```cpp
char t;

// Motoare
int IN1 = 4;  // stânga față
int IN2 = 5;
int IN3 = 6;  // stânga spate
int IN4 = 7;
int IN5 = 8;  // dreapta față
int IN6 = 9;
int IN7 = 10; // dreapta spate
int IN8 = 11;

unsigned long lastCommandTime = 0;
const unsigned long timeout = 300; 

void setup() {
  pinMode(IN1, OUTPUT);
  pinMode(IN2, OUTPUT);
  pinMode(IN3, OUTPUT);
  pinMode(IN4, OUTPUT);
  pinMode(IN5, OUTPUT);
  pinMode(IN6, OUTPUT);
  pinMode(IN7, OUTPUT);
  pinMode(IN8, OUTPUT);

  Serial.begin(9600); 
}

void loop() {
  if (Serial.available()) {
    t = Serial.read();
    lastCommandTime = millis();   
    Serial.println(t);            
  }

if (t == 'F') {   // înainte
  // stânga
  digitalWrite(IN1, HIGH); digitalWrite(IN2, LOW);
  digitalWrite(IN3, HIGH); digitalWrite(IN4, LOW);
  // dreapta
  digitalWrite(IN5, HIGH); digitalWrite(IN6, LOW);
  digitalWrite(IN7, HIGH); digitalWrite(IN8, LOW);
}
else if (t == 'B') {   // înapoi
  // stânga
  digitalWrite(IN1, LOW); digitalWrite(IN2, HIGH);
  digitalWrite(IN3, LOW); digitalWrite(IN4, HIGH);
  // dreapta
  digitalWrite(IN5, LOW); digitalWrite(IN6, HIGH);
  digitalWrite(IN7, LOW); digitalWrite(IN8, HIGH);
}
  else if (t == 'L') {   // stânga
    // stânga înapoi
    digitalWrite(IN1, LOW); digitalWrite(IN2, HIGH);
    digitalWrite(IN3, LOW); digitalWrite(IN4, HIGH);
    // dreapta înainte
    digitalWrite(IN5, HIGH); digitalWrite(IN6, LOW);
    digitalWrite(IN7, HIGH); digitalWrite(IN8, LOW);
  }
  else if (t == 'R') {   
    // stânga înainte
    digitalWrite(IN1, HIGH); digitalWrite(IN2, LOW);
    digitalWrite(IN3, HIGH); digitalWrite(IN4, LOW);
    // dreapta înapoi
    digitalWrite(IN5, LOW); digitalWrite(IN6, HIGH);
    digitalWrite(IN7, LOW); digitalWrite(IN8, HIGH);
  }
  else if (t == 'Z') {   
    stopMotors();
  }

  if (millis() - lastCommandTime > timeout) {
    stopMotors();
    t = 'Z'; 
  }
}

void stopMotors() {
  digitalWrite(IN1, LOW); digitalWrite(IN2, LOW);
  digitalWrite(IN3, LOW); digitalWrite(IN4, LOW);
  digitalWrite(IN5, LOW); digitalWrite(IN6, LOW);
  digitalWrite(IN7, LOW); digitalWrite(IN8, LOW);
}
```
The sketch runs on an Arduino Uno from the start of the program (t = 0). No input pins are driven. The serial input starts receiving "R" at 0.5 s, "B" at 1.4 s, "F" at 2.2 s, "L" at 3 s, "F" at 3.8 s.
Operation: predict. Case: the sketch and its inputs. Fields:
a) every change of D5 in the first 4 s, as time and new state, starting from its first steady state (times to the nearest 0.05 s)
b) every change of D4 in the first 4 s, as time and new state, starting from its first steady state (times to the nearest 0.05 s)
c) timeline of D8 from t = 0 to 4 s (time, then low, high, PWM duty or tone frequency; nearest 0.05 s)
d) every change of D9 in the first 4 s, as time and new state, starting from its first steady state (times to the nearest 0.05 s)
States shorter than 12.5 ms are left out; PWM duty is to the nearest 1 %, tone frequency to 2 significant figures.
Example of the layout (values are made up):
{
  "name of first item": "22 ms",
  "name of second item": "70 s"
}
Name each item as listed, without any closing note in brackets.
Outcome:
{
  "every change of D5 in the first 4 s, as time and new state, starting from its first steady state": "0 s low; 1.4 s high; 1.7 s low; 3 s high; 3.3 s low",
  "every change of D4 in the first 4 s, as time and new state, starting from its first steady state": "0 s low; 0.5 s high; 0.8 s low; 2.2 s high; 2.5 s low; 3.8 s high",
  "timeline of D8 from t = 0 to 4 s": "0 s low; 2.2 s high; 2.5 s low; 3 s high; 3.3 s low; 3.8 s high",
  "every change of D9 in the first 4 s, as time and new state, starting from its first steady state": "0 s low; 0.5 s high; 0.8 s low; 1.4 s high; 1.7 s low"
}
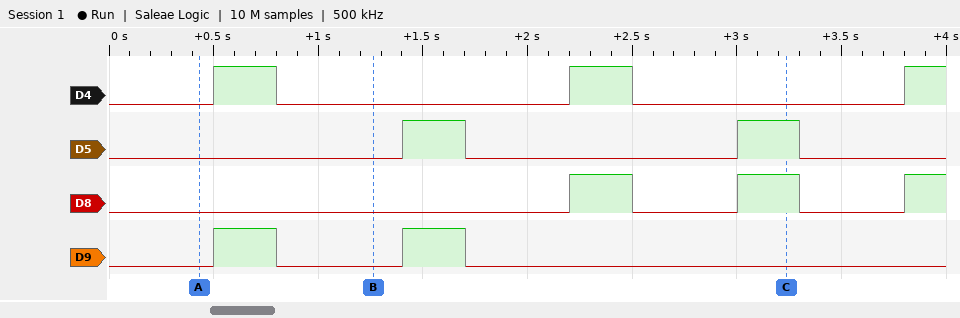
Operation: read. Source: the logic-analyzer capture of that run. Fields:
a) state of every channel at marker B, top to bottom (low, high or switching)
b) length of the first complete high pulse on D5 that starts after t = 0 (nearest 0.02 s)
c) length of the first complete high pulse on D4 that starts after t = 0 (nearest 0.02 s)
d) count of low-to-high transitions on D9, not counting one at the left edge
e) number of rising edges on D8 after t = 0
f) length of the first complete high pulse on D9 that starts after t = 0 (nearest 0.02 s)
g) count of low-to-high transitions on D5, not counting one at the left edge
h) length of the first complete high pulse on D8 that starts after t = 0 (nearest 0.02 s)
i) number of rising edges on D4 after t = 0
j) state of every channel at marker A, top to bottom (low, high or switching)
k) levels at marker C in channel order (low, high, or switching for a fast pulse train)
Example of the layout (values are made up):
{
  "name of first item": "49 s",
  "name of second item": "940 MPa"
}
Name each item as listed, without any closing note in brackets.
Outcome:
{
  "state of every channel at marker B, top to bottom": "D4 low, D5 low, D8 low, D9 low",
  "length of the first complete high pulse on D5 that starts after t = 0": "0.30 s",
  "length of the first complete high pulse on D4 that starts after t = 0": "0.30 s",
  "count of low-to-high transitions on D9, not counting one at the left edge": "2",
  "number of rising edges on D8 after t = 0": "3",
  "length of the first complete high pulse on D9 that starts after t = 0": "0.30 s",
  "count of low-to-high transitions on D5, not counting one at the left edge": "2",
  "length of the first complete high pulse on D8 that starts after t = 0": "0.30 s",
  "number of rising edges on D4 after t = 0": "3",
  "state of every channel at marker A, top to bottom": "D4 low, D5 low, D8 low, D9 low",
  "levels at marker C in channel order": "D4 low, D5 high, D8 high, D9 low"
}
